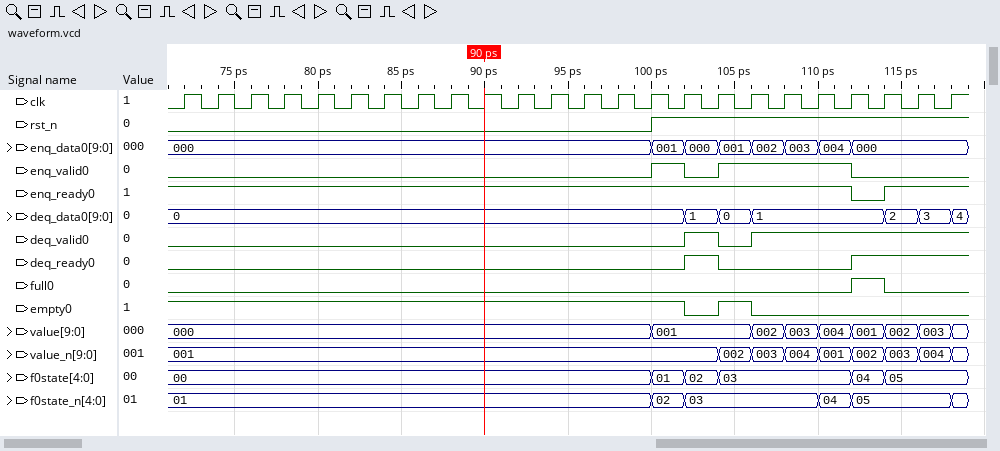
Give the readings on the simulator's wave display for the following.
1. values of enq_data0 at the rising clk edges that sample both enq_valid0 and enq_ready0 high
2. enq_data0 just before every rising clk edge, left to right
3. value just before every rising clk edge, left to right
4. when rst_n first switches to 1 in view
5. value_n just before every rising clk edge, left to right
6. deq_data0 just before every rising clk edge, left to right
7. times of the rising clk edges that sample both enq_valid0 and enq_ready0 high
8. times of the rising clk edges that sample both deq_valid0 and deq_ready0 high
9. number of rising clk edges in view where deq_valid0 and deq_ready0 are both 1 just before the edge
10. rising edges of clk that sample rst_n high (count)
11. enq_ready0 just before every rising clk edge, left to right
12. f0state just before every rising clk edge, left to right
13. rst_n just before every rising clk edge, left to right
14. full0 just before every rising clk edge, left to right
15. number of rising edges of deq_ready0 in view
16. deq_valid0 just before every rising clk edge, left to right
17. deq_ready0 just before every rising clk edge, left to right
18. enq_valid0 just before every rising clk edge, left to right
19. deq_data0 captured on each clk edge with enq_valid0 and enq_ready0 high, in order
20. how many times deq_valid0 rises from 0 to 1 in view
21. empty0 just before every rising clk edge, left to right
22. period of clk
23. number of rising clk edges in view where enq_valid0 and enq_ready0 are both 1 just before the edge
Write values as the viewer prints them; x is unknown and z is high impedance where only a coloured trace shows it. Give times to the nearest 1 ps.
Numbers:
001, 001, 002, 003, 004
000, 000, 000, 000, 000, 000, 000, 000, 000, 000, 000, 000, 000, 000, 000, 001, 000, 001, 002, 003, 004, 000, 000, 000
000, 000, 000, 000, 000, 000, 000, 000, 000, 000, 000, 000, 000, 000, 000, 001, 001, 001, 002, 003, 004, 001, 002, 003
100 ps
001, 001, 001, 001, 001, 001, 001, 001, 001, 001, 001, 001, 001, 001, 001, 001, 001, 002, 003, 004, 001, 002, 003, 004
0, 0, 0, 0, 0, 0, 0, 0, 0, 0, 0, 0, 0, 0, 0, 0, 1, 0, 1, 1, 1, 1, 2, 3
102 ps, 106 ps, 108 ps, 110 ps, 112 ps
104 ps, 114 ps, 116 ps, 118 ps
4
9
1 1 1 1 1 1 1 1 1 1 1 1 1 1 1 1 1 1 1 1 1 0 1 1
00, 00, 00, 00, 00, 00, 00, 00, 00, 00, 00, 00, 00, 00, 00, 01, 02, 03, 03, 03, 03, 04, 05, 05
0 0 0 0 0 0 0 0 0 0 0 0 0 0 0 1 1 1 1 1 1 1 1 1
0 0 0 0 0 0 0 0 0 0 0 0 0 0 0 0 0 0 0 0 0 1 0 0
2
0 0 0 0 0 0 0 0 0 0 0 0 0 0 0 0 1 0 1 1 1 1 1 1
0 0 0 0 0 0 0 0 0 0 0 0 0 0 0 0 1 0 0 0 0 1 1 1
0 0 0 0 0 0 0 0 0 0 0 0 0 0 0 1 0 1 1 1 1 0 0 0
0, 0, 1, 1, 1
2
1 1 1 1 1 1 1 1 1 1 1 1 1 1 1 1 0 1 0 0 0 0 0 0
2 ps
5
